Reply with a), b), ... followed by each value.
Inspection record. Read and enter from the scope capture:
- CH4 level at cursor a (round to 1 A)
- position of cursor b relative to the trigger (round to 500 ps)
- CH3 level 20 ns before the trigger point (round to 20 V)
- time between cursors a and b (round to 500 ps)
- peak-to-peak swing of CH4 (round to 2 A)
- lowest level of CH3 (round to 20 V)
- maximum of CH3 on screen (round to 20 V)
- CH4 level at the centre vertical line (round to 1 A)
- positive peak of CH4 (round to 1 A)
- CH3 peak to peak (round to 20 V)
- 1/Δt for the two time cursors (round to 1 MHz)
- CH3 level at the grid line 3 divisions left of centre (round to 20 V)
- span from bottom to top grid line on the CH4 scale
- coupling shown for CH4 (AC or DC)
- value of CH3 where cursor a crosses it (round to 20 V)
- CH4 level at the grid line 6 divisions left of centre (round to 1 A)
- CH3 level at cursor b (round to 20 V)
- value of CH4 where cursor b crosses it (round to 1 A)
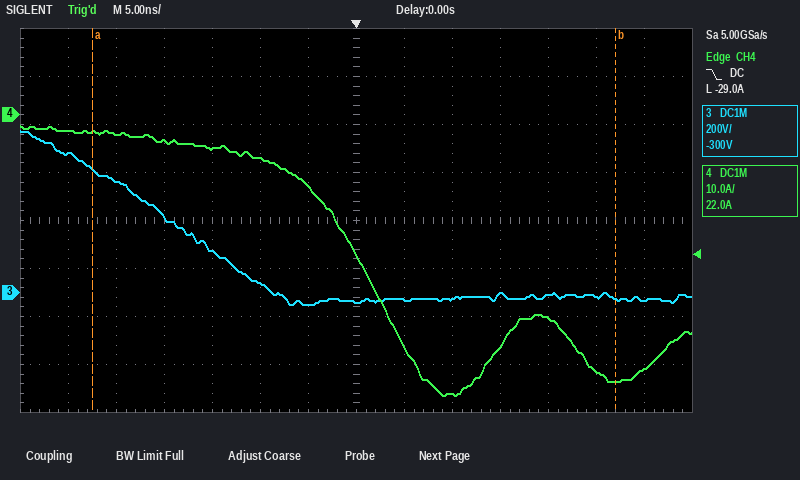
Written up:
a) -3 A
b) +27.0 ns
c) 320 V
d) 54.5 ns
e) 56 A
f) -40 V
g) 680 V
h) -29 A
i) -2 A
j) 720 V
k) 18 MHz
l) 180 V
m) 80 A
n) DC
o) 520 V
p) -3 A
q) -20 V
r) -56 A
